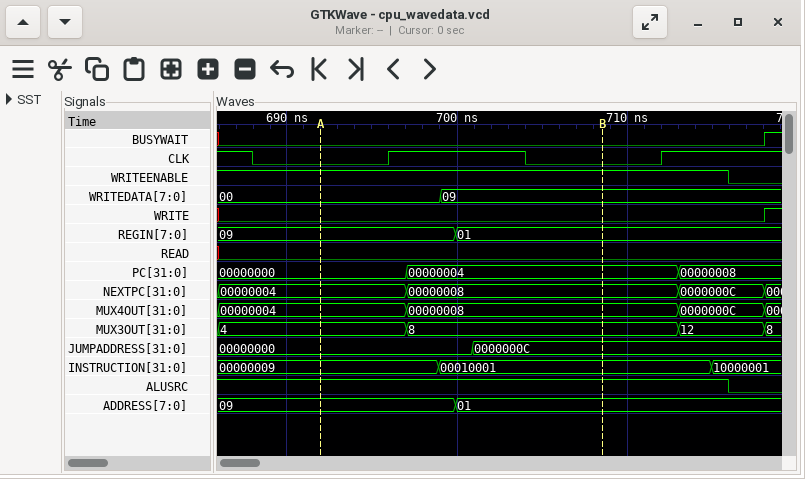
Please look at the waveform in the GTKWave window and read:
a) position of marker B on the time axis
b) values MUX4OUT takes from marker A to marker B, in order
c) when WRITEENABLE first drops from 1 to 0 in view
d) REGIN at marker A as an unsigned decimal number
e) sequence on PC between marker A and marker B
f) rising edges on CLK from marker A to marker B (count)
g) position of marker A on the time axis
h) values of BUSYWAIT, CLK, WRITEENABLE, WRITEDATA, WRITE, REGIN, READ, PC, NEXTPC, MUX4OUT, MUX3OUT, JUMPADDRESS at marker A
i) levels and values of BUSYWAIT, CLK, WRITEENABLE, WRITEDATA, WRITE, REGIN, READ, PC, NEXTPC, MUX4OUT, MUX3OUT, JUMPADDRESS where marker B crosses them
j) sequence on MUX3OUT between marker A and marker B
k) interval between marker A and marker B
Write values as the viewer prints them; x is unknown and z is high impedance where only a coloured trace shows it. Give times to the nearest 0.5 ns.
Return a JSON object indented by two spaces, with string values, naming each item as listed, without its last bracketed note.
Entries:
{
  "position of marker B on the time axis": "708.5 ns",
  "values MUX4OUT takes from marker A to marker B, in order": "00000004, 00000008",
  "when WRITEENABLE first drops from 1 to 0 in view": "716 ns",
  "REGIN at marker A as an unsigned decimal number": "9",
  "sequence on PC between marker A and marker B": "00000000, 00000004",
  "rising edges on CLK from marker A to marker B": "1",
  "position of marker A on the time axis": "692 ns",
  "values of BUSYWAIT, CLK, WRITEENABLE, WRITEDATA, WRITE, REGIN, READ, PC, NEXTPC, MUX4OUT, MUX3OUT, JUMPADDRESS at marker A": "BUSYWAIT=0, CLK=0, WRITEENABLE=1, WRITEDATA=00, WRITE=0, REGIN=09, READ=0, PC=00000000, NEXTPC=00000004, MUX4OUT=00000004, MUX3OUT=4, JUMPADDRESS=00000000",
  "levels and values of BUSYWAIT, CLK, WRITEENABLE, WRITEDATA, WRITE, REGIN, READ, PC, NEXTPC, MUX4OUT, MUX3OUT, JUMPADDRESS where marker B crosses them": "BUSYWAIT=0, CLK=0, WRITEENABLE=1, WRITEDATA=09, WRITE=0, REGIN=01, READ=0, PC=00000004, NEXTPC=00000008, MUX4OUT=00000008, MUX3OUT=8, JUMPADDRESS=0000000C",
  "sequence on MUX3OUT between marker A and marker B": "4, 8",
  "interval between marker A and marker B": "16.5 ns"
}
